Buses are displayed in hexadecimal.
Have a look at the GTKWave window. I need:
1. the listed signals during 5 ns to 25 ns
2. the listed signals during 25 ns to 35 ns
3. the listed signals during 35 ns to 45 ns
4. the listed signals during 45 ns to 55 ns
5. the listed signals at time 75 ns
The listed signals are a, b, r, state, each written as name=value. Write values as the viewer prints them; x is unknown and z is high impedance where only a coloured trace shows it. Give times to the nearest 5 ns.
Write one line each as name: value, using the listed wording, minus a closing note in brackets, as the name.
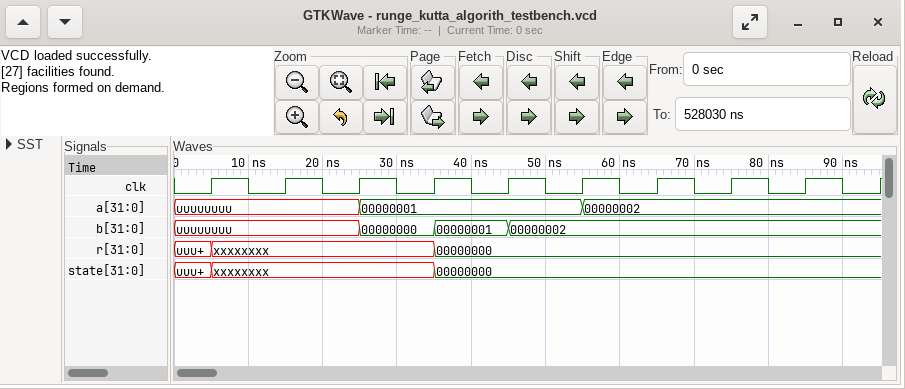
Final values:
the listed signals during 5 ns to 25 ns: a=uuuuuuuu, b=uuuuuuuu, r=xxxxxxxx, state=xxxxxxxx
the listed signals during 25 ns to 35 ns: a=00000001, b=00000000, r=xxxxxxxx, state=xxxxxxxx
the listed signals during 35 ns to 45 ns: a=00000001, b=00000001, r=00000000, state=00000000
the listed signals during 45 ns to 55 ns: a=00000001, b=00000002, r=00000000, state=00000000
the listed signals at time 75 ns: a=00000002, b=00000002, r=00000000, state=00000000
